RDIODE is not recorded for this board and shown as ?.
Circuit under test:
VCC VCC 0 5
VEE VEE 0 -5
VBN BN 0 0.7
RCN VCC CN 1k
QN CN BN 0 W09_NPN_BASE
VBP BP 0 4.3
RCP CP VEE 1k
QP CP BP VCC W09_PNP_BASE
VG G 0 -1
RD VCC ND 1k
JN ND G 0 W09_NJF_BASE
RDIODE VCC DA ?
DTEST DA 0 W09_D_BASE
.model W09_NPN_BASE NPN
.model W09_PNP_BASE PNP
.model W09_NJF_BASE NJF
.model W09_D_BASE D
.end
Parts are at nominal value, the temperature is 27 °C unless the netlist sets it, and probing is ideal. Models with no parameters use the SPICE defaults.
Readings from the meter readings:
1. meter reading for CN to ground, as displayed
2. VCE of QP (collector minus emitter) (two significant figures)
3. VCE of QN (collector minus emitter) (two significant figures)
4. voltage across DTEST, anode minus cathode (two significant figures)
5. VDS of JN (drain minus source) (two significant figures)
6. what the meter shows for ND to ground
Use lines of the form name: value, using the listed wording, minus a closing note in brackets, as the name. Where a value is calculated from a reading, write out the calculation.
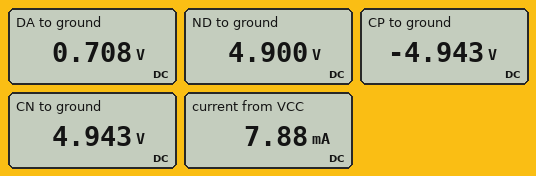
meter reading for CN to ground, as displayed: 4.943 V
VCE of QP (collector minus emitter): -4.943 V - 5 V = -9.9 V
VCE of QN (collector minus emitter): 4.943 V = 4.9 V
voltage across DTEST, anode minus cathode: 708 mV = 710 mV
VDS of JN (drain minus source): 4.9 V = 4.9 V
what the meter shows for ND to ground: 4.900 V
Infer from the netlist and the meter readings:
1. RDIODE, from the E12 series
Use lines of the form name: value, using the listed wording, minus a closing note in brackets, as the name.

RDIODE, from the E12 series: 560 Ω
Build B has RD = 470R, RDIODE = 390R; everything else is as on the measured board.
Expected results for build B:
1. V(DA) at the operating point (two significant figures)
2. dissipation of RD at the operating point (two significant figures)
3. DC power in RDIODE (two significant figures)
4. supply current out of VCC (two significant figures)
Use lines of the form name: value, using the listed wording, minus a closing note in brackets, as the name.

V(DA) at the operating point: 720 mV
dissipation of RD at the operating point: 4.7 µW
DC power in RDIODE: 47 mW
supply current out of VCC: 11 mA
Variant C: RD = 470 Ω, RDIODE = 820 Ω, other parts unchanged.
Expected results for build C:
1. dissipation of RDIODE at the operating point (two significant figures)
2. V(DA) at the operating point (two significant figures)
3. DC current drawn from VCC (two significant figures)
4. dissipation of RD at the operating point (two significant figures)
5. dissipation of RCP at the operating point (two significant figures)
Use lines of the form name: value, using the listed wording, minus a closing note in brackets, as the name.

dissipation of RDIODE at the operating point: 23 mW
V(DA) at the operating point: 700 mV
DC current drawn from VCC: 5.5 mA
dissipation of RD at the operating point: 4.7 µW
dissipation of RCP at the operating point: 3.2 µW
